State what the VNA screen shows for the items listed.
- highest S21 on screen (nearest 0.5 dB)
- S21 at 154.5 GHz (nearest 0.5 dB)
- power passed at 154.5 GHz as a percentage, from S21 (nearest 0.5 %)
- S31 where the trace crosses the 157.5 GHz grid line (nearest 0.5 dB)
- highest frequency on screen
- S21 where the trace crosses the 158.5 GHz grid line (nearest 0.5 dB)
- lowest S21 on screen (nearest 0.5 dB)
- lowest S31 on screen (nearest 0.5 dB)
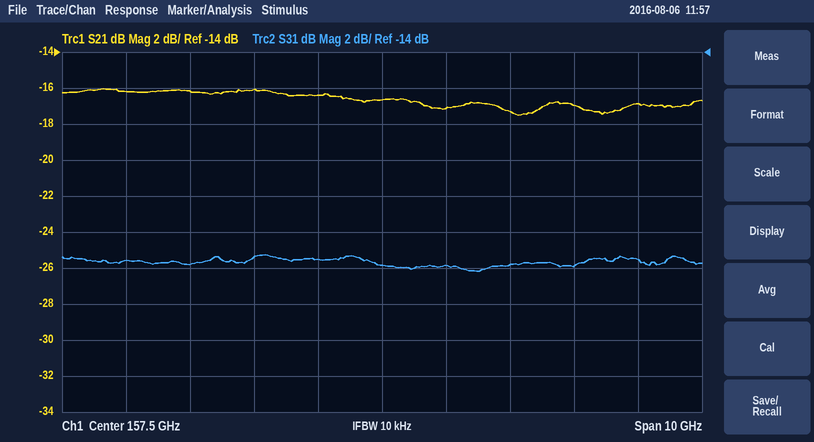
-16.0 dB
-16.0 dB
2.5 %
-26.0 dB
162.5 GHz
-17.0 dB
-17.5 dB
-26.0 dB
